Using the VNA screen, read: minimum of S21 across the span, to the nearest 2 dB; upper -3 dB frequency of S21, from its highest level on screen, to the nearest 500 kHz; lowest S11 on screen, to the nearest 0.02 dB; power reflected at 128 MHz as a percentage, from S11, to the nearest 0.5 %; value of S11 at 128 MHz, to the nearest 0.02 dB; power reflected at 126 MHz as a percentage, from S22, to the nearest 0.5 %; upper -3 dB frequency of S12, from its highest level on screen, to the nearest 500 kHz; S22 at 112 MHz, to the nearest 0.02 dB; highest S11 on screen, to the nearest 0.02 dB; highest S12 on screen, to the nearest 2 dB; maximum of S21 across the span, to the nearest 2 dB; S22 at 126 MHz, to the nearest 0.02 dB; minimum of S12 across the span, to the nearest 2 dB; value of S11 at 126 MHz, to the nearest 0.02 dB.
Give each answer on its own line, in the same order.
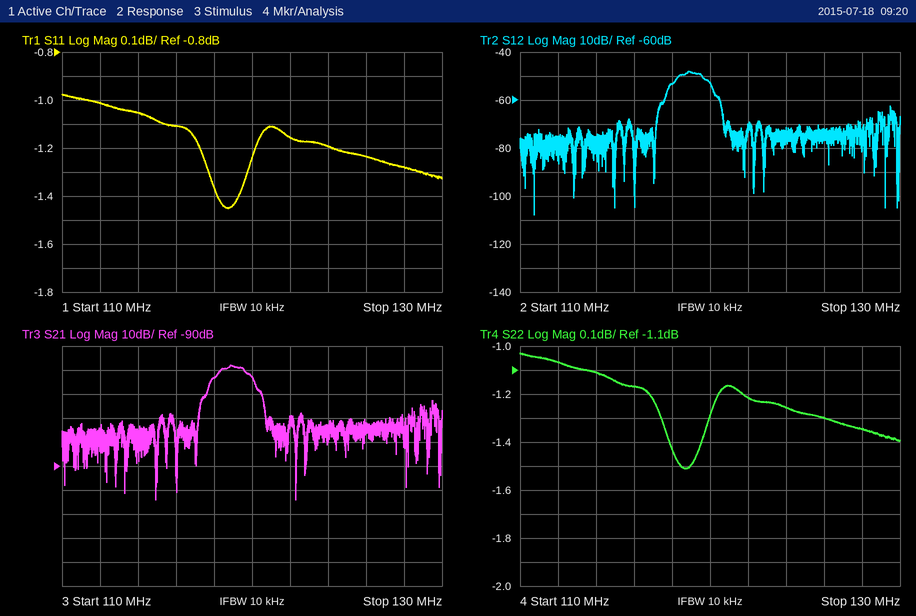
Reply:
-104 dB
119.5 MHz
-1.46 dB
74.5 %
-1.28 dB
74.0 %
119.5 MHz
-1.06 dB
-0.98 dB
-48 dB
-48 dB
-1.30 dB
-108 dB
-1.24 dB
